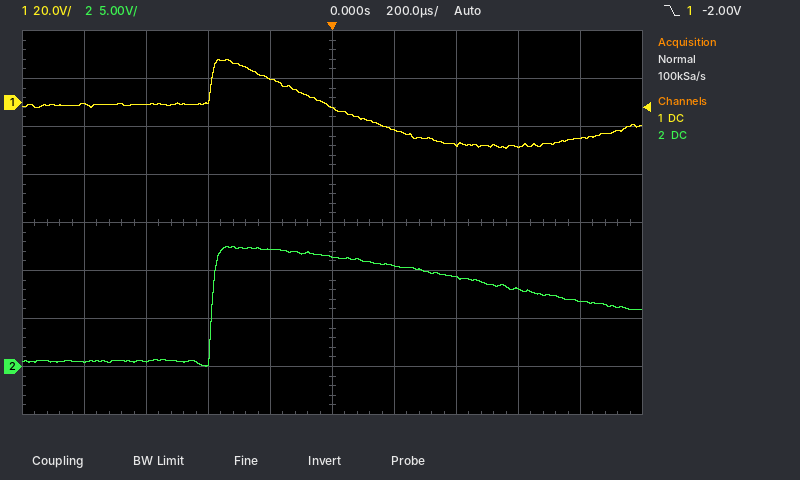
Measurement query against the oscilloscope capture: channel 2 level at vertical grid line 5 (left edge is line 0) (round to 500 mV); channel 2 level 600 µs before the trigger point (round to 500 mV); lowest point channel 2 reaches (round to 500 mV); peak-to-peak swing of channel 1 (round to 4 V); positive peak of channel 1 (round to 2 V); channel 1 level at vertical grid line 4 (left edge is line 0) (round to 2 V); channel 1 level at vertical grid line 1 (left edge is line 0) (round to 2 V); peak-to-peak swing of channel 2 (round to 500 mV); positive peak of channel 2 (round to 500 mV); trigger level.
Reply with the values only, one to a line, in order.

11.5 V
500 mV
0.0 V
36 V
18 V
10 V
0 V
12.5 V
12.5 V
-2.00 V
